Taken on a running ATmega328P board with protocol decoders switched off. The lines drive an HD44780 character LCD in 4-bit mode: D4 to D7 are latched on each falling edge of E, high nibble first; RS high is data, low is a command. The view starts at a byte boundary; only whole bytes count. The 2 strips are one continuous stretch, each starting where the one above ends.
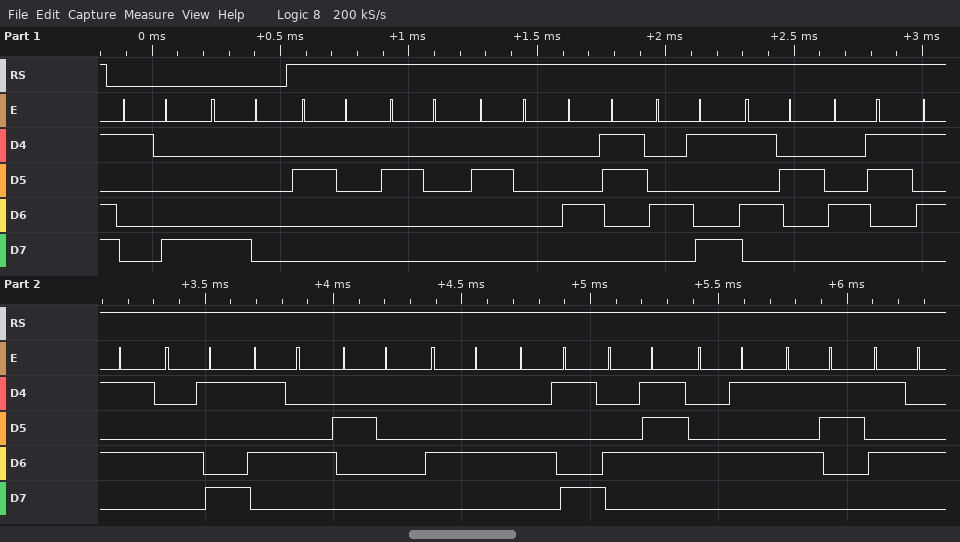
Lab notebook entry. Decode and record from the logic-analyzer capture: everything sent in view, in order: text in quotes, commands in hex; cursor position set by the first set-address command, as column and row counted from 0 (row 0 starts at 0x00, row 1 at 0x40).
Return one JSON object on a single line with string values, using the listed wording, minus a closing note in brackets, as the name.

{"everything sent in view, in order: text in quotes, commands in hex": "0x18 0x80 \"   CIRCUIT DIGEST\"", "cursor position set by the first set-address command, as column and row counted from 0": "column 0, row 0"}
